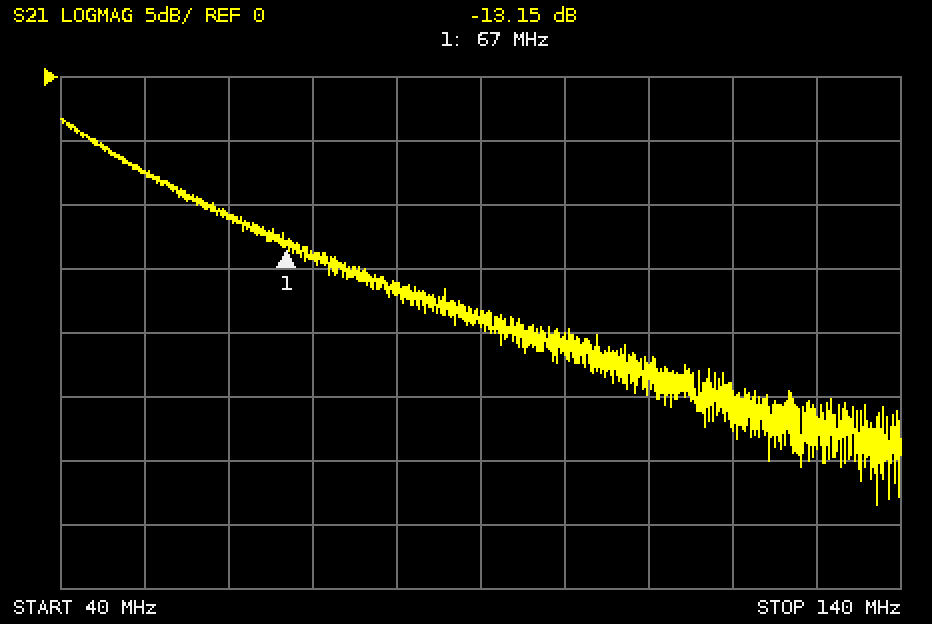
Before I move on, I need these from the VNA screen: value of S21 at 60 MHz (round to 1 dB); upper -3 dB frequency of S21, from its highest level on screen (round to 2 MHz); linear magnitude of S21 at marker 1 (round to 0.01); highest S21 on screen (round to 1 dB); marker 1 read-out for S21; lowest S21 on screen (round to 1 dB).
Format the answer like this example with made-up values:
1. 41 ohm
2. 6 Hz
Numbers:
1. -11 dB
2. 46 MHz
3. 0.22
4. -3 dB
5. -13.15 dB
6. -33 dB
